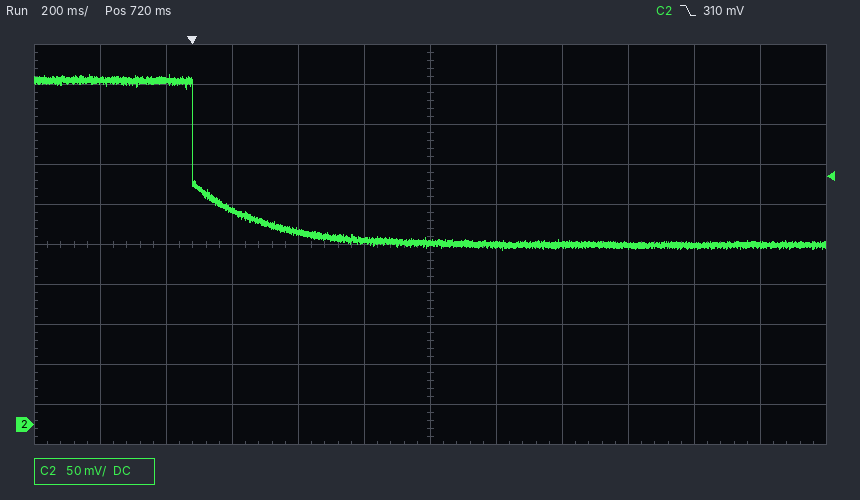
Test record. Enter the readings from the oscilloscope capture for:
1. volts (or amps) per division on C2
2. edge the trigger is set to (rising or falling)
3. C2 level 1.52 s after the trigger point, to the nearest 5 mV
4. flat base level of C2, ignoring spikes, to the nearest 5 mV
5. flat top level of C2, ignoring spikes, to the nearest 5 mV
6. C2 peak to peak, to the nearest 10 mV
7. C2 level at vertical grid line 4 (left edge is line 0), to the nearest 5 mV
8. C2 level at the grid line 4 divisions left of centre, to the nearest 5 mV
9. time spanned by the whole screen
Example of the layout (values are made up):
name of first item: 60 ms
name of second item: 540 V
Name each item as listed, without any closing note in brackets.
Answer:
volts (or amps) per division on C2: 50 mV
edge the trigger is set to: falling
C2 level 1.52 s after the trigger point, to the nearest 5 mV: 225 mV
flat base level of C2, ignoring spikes, to the nearest 5 mV: 225 mV
flat top level of C2, ignoring spikes, to the nearest 5 mV: 430 mV
C2 peak to peak, to the nearest 10 mV: 220 mV
C2 level at vertical grid line 4 (left edge is line 0), to the nearest 5 mV: 240 mV
C2 level at the grid line 4 divisions left of centre, to the nearest 5 mV: 430 mV
time spanned by the whole screen: 2.4 s
